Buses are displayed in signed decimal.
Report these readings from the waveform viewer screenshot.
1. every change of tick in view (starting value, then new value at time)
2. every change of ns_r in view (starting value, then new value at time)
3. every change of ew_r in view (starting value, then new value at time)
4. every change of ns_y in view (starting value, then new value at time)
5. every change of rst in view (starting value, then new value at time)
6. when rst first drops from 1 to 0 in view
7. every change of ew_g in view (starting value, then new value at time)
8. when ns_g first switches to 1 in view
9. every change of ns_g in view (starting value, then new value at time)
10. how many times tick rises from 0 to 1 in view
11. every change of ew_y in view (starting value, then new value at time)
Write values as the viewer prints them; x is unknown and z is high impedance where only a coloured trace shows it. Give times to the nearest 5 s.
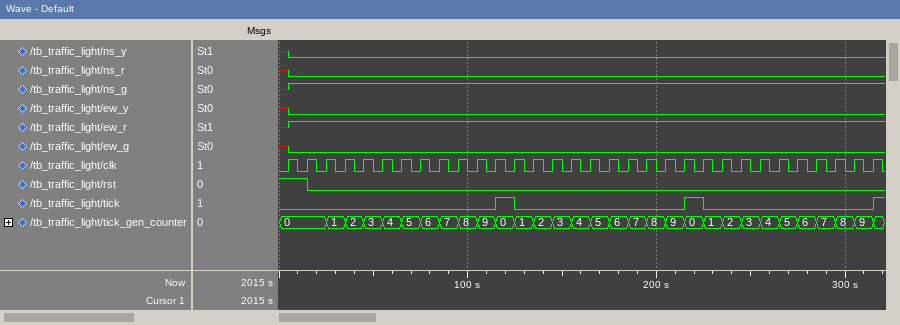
0, 1 at 115 s, 0 at 125 s, 1 at 215 s, 0 at 225 s, 1 at 315 s
x, 0 at 5 s
x, 1 at 5 s
x, 0 at 5 s
1, 0 at 15 s
15 s
x, 0 at 5 s
5 s
x, 1 at 5 s
3
x, 0 at 5 s
